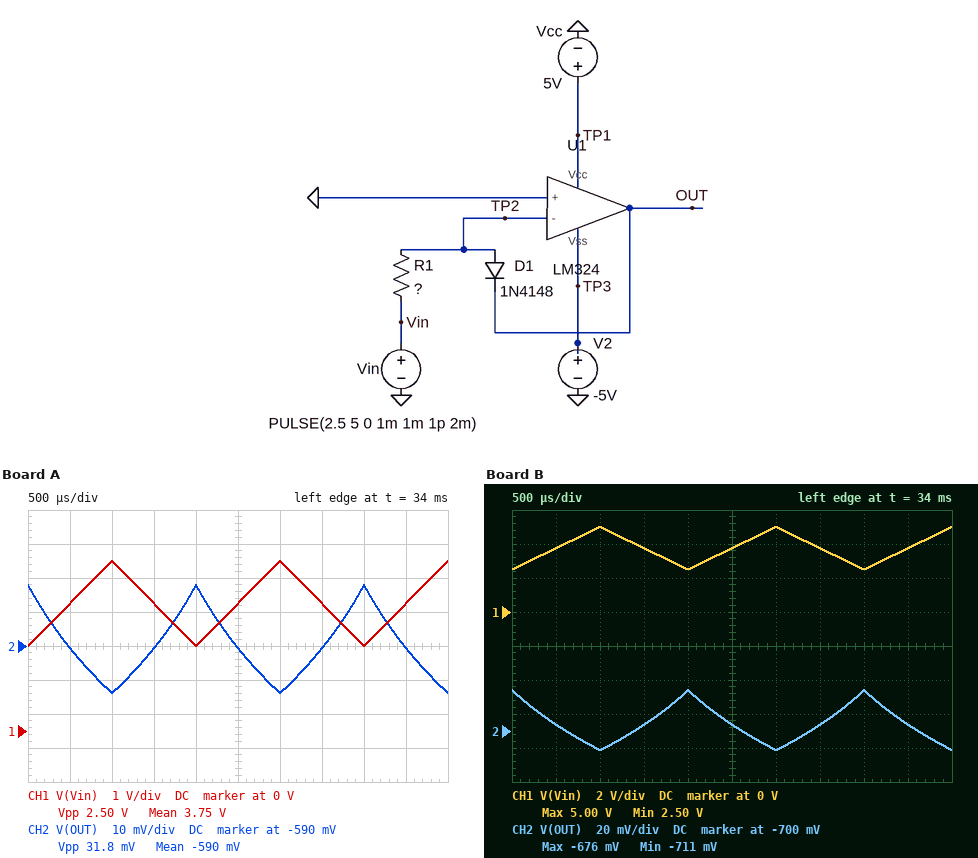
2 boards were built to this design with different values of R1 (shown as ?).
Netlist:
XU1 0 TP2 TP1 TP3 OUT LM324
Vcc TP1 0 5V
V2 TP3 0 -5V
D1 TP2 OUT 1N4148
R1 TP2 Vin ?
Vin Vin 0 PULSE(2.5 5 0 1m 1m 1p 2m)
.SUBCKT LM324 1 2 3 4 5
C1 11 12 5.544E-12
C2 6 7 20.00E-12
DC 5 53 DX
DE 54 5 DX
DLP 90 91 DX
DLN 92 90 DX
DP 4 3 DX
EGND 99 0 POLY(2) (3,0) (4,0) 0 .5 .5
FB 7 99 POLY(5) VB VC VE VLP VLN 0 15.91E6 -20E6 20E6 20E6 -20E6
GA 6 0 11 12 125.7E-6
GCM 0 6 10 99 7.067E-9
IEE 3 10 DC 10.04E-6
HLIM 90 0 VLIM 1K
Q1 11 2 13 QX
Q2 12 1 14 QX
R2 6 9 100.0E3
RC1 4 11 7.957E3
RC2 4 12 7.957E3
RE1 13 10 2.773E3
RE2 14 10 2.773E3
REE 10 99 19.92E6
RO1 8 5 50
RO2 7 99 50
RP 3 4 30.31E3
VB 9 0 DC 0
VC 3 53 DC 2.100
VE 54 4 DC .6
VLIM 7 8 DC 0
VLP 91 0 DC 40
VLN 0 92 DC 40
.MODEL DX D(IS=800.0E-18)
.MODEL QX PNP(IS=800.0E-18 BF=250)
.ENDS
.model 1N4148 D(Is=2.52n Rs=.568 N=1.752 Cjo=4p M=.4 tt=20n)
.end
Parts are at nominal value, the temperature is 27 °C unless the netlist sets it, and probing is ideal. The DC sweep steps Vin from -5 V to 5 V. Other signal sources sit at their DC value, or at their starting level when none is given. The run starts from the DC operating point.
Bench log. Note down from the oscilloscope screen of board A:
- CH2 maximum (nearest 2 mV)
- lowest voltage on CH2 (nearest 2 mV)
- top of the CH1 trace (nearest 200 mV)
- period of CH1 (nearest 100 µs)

-572 mV
-604 mV
5.0 V
2.0 ms
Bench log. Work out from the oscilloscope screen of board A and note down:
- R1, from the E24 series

3.3 kΩ
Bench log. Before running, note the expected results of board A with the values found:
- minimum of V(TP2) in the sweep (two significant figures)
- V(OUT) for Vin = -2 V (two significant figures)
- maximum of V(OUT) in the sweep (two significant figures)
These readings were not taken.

-5.0 V
3.5 V
3.5 V
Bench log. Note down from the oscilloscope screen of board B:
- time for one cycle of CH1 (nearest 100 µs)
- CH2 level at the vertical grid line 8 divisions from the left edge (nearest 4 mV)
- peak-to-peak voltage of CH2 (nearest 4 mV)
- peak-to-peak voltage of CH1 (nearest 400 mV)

2.0 ms
-676 mV
36 mV
2.4 V
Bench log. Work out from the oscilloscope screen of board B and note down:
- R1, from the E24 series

360 Ω
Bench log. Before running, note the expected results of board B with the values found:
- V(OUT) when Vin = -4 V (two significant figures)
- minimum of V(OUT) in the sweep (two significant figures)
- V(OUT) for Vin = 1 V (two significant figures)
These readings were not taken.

3.5 V
-710 mV
-630 mV
